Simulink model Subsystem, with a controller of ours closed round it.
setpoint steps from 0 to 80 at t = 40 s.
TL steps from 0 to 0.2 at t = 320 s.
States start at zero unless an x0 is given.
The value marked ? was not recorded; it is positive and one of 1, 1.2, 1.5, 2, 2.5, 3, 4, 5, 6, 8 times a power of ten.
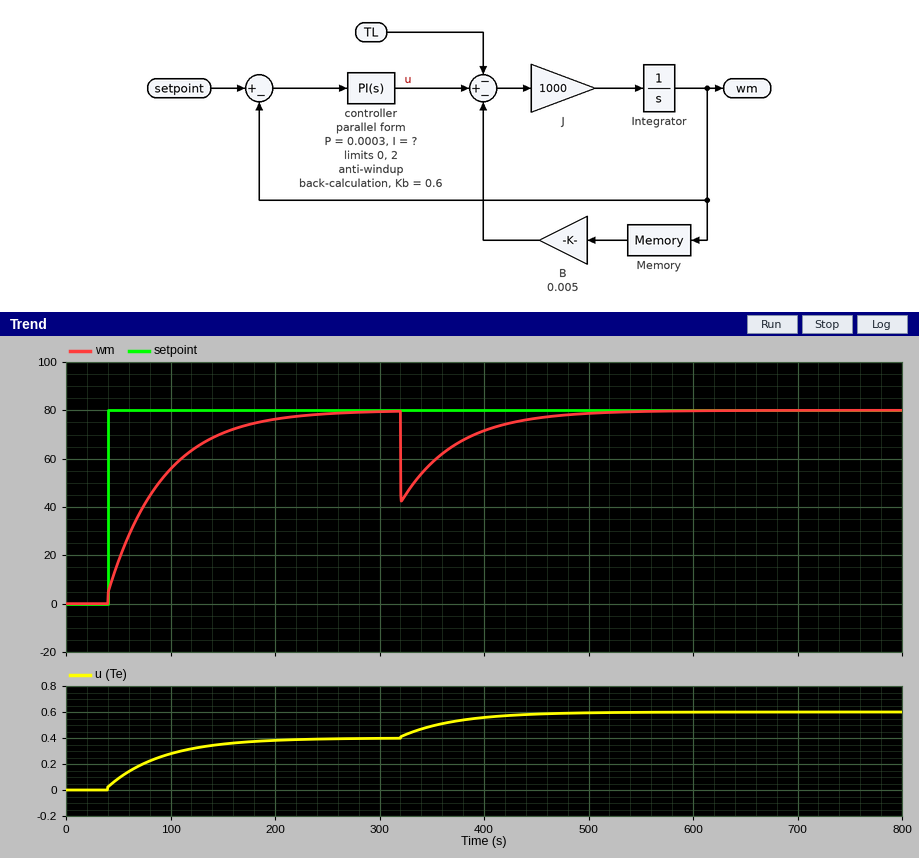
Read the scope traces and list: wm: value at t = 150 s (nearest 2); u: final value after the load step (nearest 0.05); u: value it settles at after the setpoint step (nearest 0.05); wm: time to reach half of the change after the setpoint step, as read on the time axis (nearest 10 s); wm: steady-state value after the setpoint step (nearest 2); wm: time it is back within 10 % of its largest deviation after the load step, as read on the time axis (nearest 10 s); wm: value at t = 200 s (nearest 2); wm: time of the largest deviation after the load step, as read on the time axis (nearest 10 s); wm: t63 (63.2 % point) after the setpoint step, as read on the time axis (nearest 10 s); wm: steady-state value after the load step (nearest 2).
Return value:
70
0.60
0.40
70 s
80
440 s
76
320 s
90 s
80
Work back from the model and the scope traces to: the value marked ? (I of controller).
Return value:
0.0001
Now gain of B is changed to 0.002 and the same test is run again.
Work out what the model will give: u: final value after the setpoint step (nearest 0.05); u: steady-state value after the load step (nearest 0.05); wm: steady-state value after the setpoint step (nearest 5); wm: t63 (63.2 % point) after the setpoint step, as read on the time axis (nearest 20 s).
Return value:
0.15
0.35
80
60 s
